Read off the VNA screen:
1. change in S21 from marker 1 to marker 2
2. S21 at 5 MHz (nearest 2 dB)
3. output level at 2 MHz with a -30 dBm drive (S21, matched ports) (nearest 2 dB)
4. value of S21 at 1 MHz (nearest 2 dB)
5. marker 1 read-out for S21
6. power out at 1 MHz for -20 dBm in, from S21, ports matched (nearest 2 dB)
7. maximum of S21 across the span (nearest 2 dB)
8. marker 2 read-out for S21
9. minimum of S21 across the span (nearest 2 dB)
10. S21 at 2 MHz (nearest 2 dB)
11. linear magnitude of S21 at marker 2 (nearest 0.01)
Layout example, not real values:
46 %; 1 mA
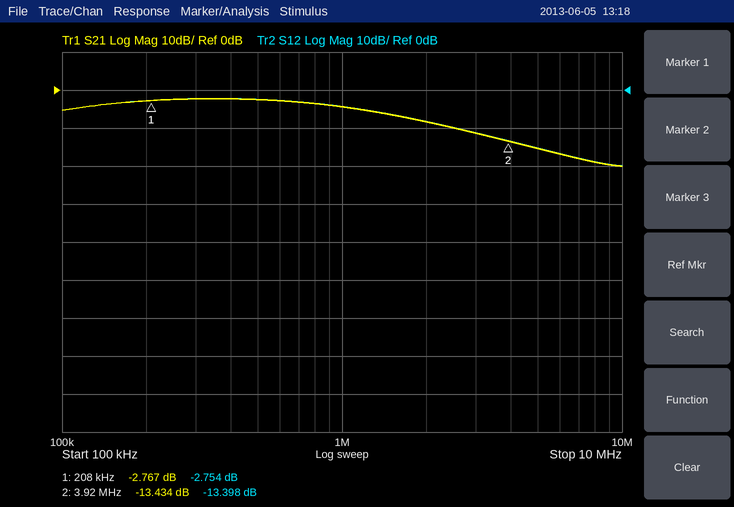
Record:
-10.667 dB; -16 dB; -38 dBm; -4 dB; -2.767 dB; -24 dBm; -2 dB; -13.434 dB; -20 dB; -8 dB; 0.21
